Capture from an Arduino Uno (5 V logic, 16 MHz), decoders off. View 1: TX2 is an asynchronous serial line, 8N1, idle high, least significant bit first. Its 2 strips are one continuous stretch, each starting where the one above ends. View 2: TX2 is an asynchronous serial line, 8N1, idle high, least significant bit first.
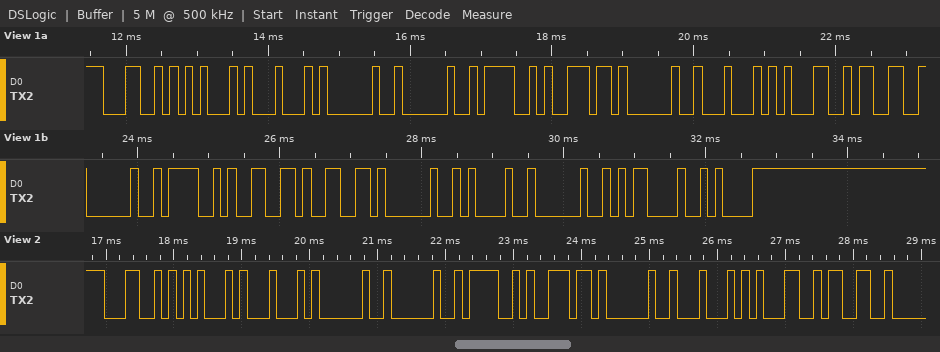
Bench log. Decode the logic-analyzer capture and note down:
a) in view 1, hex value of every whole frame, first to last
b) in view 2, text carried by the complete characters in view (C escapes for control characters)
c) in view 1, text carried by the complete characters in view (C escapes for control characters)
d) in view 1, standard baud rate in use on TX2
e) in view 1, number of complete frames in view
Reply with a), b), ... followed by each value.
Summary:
a) 4C 45 44 20 20 4F 6E 20 44 31 33 20 4F 66 66 20 21 20 0D 0A
b) "LED  On D13"
c) "LED  On D13 Off ! \r\n"
d) 9600 baud
e) 20
